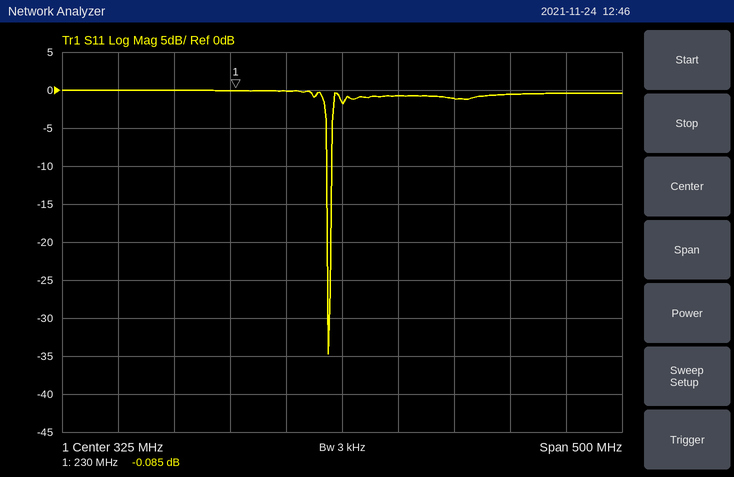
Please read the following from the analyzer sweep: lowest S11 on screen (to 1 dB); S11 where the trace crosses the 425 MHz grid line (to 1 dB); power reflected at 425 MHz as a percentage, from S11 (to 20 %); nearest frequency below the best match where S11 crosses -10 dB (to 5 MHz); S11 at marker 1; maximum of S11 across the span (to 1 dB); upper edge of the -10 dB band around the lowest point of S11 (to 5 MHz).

-35 dB
-1 dB
80 %
310 MHz
-0.085 dB
0 dB
315 MHz
